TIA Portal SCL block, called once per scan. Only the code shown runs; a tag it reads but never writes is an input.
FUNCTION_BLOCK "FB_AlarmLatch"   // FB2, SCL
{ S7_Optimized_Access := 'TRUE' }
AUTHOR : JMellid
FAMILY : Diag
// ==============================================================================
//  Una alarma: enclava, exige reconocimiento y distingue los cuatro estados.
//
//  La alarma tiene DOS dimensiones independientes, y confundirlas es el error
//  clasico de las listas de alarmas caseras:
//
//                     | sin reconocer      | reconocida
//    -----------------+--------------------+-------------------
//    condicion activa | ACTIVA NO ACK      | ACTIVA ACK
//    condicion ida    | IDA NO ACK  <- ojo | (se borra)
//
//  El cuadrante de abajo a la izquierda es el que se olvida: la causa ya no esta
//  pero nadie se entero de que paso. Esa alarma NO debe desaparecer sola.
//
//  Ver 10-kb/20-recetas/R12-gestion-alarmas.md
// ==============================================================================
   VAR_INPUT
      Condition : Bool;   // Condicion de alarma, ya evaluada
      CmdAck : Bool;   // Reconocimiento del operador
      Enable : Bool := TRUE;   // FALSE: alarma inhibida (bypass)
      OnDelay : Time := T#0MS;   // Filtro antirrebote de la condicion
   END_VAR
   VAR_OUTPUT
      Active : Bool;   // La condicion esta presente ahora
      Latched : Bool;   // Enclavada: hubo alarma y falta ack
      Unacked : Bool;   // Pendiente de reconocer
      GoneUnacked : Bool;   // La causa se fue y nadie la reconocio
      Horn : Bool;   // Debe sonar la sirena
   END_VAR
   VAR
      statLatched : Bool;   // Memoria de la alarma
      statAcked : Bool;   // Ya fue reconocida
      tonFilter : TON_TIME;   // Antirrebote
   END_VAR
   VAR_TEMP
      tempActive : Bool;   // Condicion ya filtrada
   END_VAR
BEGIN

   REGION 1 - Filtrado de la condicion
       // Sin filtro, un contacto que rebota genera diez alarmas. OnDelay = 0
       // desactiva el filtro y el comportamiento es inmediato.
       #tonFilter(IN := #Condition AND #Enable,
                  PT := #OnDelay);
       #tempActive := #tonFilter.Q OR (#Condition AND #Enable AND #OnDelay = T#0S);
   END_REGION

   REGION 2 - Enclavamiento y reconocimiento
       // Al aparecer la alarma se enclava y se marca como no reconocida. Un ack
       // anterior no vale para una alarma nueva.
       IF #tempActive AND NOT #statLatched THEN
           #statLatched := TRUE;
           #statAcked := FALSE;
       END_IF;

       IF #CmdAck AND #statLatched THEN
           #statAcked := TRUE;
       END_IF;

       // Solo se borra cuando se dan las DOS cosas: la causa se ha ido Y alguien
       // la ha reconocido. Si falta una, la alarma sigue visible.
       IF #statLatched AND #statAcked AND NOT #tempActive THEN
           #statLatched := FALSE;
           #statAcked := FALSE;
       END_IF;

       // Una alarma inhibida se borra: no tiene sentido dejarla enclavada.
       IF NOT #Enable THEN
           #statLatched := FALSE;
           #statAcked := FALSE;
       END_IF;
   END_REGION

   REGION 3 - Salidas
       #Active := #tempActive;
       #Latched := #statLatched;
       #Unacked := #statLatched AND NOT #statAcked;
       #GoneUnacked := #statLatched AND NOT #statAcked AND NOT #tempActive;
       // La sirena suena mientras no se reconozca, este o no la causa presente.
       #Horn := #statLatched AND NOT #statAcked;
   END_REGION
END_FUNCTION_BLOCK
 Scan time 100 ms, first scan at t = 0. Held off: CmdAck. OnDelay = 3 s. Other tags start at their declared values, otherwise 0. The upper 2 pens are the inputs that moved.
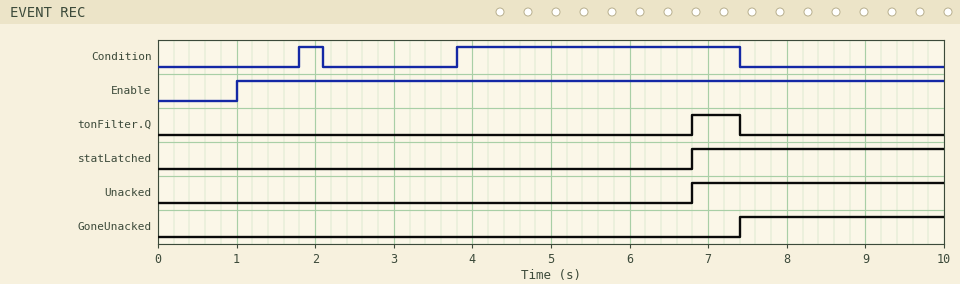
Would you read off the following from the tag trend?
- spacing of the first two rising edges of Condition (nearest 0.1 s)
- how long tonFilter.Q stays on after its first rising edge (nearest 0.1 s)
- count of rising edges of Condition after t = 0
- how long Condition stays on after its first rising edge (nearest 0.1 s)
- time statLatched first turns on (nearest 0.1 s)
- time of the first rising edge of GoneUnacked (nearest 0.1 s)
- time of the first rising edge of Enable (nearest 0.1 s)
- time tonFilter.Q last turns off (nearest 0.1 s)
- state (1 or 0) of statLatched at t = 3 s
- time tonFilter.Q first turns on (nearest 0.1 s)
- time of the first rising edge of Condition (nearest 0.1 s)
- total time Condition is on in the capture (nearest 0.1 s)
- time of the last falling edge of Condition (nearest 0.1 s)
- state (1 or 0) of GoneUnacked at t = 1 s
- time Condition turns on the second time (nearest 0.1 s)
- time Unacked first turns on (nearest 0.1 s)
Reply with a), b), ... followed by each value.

a) 2.0 s
b) 0.6 s
c) 2
d) 0.3 s
e) 6.8 s
f) 7.4 s
g) 1.0 s
h) 7.4 s
i) 0
j) 6.8 s
k) 1.8 s
l) 3.9 s
m) 7.4 s
n) 0
o) 3.8 s
p) 6.8 s
